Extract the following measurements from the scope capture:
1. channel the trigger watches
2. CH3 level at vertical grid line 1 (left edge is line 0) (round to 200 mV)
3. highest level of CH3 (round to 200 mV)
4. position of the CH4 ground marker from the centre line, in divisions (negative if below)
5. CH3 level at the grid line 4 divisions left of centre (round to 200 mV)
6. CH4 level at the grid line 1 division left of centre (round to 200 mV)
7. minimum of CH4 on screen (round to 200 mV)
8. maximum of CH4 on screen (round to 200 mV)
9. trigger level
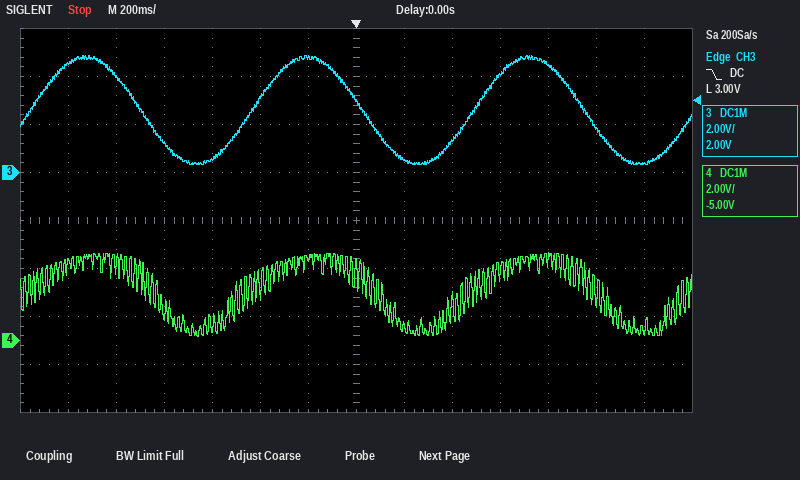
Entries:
CH3
4.6 V
4.8 V
-2.5 div
1.2 V
3.4 V
200 mV
3.6 V
3.00 V
